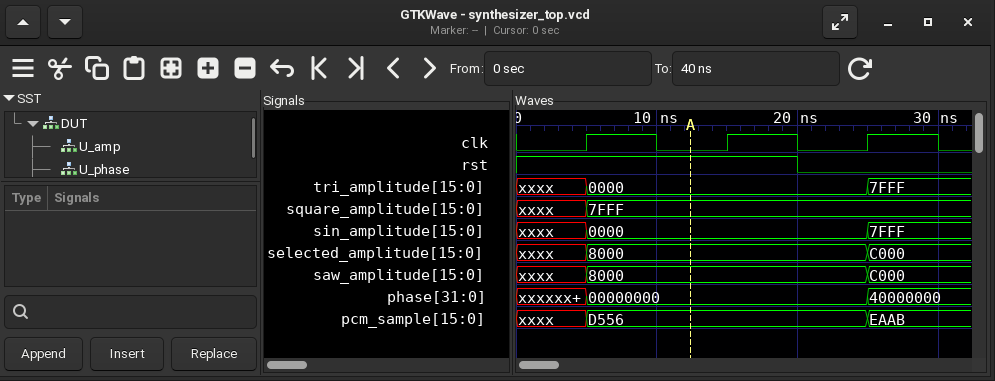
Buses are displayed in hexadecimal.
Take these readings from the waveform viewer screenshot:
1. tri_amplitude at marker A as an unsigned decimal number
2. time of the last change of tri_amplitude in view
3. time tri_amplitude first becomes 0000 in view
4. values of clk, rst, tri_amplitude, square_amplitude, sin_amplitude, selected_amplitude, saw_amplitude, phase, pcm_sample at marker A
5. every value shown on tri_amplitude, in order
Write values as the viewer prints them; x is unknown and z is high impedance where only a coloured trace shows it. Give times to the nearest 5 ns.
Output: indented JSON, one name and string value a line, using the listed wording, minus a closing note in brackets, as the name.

{
  "tri_amplitude at marker A as an unsigned decimal number": "0",
  "time of the last change of tri_amplitude in view": "25 ns",
  "time tri_amplitude first becomes 0000 in view": "5 ns",
  "values of clk, rst, tri_amplitude, square_amplitude, sin_amplitude, selected_amplitude, saw_amplitude, phase, pcm_sample at marker A": "clk=0, rst=1, tri_amplitude=0000, square_amplitude=7FFF, sin_amplitude=0000, selected_amplitude=8000, saw_amplitude=8000, phase=00000000, pcm_sample=D556",
  "every value shown on tri_amplitude, in order": "xxxx, 0000, 7FFF"
}
